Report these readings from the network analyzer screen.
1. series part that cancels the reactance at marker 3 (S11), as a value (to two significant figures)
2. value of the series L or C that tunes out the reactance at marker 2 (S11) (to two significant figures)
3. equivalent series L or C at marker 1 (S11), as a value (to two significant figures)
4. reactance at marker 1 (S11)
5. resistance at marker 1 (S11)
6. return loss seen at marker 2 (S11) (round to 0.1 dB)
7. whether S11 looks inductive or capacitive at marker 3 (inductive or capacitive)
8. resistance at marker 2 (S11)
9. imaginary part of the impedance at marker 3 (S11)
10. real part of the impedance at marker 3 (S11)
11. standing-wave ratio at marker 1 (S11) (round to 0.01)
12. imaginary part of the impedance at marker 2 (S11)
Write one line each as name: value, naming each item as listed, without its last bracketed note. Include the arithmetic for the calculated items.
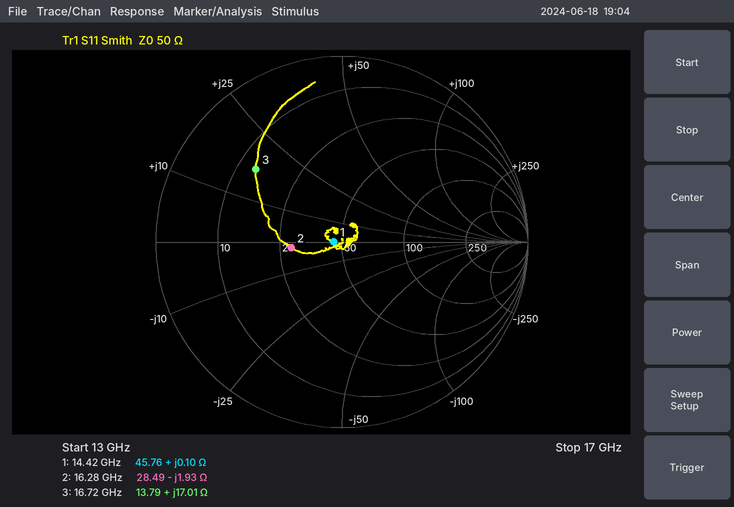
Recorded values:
series part that cancels the reactance at marker 3 (S11), as a value: C = 1/(2π × 16.72 GHz × 17.01 Ω) ≈ 560 fF
value of the series L or C that tunes out the reactance at marker 2 (S11): L = 1.93 Ω/(2π × 16.28 GHz) ≈ 19 pH
equivalent series L or C at marker 1 (S11), as a value: L = 0.1 Ω/(2π × 14.42 GHz) ≈ 1.1 pH
reactance at marker 1: +0.10 Ω
resistance at marker 1: 45.76 Ω
return loss seen at marker 2 (S11): 11.2 dB
whether S11 looks inductive or capacitive at marker 3: inductive
resistance at marker 2: 28.49 Ω
imaginary part of the impedance at marker 3: +17.01 Ω
real part of the impedance at marker 3: 13.79 Ω
standing-wave ratio at marker 1 (S11): 1.09
imaginary part of the impedance at marker 2: -1.93 Ω
